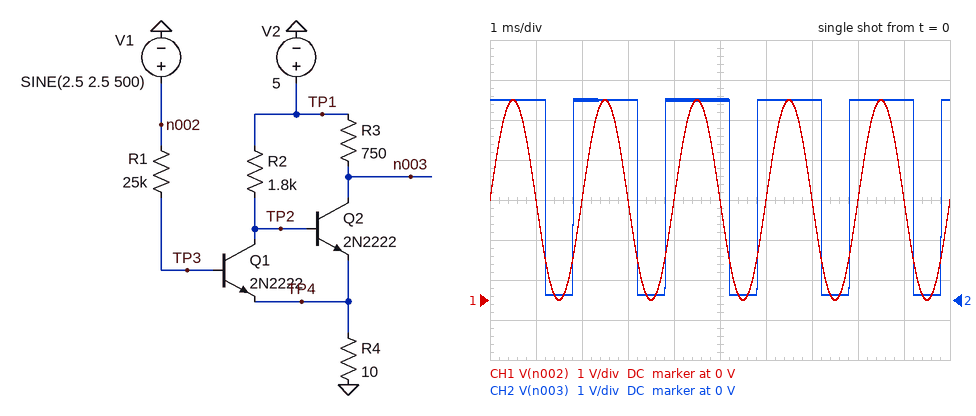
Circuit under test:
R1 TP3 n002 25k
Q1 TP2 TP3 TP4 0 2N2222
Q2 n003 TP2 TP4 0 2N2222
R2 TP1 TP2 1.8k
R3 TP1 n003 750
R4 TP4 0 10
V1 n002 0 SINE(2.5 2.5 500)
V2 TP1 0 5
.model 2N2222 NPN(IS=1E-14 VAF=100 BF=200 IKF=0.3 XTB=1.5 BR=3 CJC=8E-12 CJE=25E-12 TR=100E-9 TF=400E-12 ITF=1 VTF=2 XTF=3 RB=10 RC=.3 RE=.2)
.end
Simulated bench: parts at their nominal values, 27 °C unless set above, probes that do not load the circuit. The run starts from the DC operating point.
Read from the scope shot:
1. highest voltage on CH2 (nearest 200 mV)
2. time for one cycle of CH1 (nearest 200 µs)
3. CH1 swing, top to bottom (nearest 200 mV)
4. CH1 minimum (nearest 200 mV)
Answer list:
5.0 V
2.0 ms
5.0 V
0 V
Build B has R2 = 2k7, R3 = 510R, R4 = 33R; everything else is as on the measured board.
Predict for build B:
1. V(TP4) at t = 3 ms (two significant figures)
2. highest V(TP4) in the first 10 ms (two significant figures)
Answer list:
62 mV
350 mV
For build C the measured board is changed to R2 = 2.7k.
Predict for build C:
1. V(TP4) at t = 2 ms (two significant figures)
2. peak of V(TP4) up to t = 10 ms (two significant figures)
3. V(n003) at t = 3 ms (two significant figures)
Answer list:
19 mV
81 mV
5.0 V
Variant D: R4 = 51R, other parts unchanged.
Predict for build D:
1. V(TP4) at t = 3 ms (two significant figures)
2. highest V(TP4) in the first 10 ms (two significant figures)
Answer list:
140 mV
420 mV
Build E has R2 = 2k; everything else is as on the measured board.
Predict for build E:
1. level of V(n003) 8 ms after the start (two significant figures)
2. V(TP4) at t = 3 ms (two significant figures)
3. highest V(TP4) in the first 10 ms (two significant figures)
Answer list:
5.0 V
25 mV
86 mV
